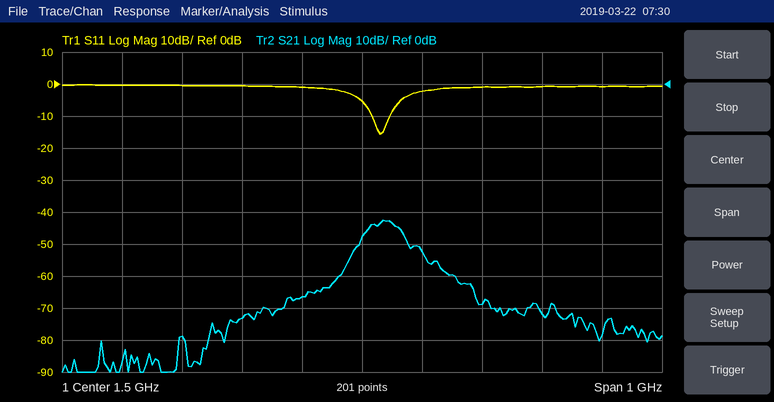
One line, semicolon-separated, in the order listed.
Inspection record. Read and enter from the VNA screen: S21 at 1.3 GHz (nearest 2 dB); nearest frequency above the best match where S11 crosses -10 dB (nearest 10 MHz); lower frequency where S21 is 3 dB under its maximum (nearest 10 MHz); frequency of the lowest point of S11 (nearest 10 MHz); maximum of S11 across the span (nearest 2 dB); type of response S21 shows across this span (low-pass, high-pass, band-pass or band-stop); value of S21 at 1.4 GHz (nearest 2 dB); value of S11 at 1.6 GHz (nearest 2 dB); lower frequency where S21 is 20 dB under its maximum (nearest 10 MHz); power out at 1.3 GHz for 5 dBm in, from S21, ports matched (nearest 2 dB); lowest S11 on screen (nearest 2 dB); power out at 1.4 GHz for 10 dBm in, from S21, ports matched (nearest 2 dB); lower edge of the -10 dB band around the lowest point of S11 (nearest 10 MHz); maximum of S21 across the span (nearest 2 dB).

-74 dB; 1.55 GHz; 1.51 GHz; 1.53 GHz; 0 dB; band-pass; -66 dB; -2 dB; 1.45 GHz; -68 dBm; -16 dB; -56 dBm; 1.52 GHz; -42 dB
